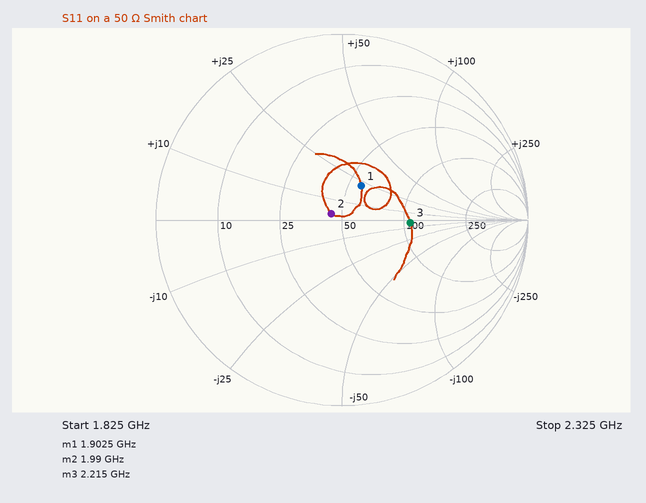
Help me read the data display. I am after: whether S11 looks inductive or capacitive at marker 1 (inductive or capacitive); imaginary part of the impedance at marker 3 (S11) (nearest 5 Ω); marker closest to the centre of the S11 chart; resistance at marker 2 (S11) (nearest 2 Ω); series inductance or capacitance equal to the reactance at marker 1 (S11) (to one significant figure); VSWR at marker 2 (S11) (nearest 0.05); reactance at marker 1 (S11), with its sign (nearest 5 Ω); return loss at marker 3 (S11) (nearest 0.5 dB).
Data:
inductive
-5 Ω
marker 2
44 Ω
2 nH
1.15
+20 Ω
8.5 dB
